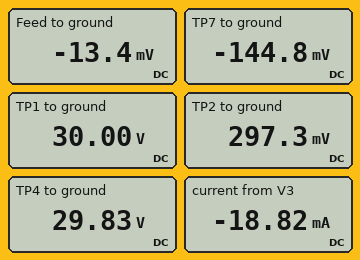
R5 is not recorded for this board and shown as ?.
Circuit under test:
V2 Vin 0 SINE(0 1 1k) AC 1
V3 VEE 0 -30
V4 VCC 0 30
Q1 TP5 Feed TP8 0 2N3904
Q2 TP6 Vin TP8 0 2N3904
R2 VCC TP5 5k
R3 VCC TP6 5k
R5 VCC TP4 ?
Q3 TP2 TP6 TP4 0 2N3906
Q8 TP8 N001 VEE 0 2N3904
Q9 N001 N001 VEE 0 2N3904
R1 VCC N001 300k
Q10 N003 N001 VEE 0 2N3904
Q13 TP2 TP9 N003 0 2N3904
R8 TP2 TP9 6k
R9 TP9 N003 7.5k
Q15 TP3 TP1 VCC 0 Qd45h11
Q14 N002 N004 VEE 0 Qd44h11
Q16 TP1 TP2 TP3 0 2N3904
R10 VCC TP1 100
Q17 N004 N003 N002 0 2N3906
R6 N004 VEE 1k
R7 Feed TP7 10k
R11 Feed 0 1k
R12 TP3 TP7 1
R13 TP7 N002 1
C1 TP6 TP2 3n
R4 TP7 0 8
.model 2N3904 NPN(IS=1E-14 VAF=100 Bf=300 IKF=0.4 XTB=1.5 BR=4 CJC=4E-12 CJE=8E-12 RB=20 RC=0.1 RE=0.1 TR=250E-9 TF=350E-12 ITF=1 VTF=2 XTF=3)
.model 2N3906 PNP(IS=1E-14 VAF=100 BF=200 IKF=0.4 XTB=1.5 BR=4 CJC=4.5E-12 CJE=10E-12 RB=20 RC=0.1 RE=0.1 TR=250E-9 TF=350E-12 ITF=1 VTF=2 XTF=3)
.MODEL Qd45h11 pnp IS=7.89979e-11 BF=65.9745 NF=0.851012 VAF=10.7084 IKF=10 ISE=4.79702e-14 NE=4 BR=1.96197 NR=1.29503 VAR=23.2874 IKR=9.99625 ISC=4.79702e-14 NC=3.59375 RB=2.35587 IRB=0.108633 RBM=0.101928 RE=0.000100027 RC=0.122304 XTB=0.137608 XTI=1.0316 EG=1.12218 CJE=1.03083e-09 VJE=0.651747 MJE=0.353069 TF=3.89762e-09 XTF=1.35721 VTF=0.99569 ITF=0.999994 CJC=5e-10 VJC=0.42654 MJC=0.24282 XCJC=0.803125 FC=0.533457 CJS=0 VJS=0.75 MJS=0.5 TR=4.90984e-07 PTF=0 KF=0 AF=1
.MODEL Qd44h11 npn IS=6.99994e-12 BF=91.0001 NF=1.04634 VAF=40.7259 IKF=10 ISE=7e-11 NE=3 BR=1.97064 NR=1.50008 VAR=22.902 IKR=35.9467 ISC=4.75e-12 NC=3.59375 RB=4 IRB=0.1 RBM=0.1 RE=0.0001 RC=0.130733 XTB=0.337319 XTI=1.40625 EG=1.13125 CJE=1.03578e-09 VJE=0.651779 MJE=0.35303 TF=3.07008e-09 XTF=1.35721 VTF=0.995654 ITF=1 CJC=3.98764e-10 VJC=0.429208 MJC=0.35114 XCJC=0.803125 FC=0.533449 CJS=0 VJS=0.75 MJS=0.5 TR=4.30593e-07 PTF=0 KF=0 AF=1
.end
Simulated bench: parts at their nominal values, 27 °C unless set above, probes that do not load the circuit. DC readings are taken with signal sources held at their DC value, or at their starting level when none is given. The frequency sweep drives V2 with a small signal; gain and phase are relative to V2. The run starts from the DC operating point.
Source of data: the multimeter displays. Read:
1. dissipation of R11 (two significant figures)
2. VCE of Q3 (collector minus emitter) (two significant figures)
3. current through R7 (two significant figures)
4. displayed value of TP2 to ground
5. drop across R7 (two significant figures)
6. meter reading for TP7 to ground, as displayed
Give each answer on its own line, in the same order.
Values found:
180 nW
-30 V
13 µA
297.3 mV
130 mV
-144.8 mV
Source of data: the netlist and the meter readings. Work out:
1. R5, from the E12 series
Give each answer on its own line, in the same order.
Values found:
680 Ω
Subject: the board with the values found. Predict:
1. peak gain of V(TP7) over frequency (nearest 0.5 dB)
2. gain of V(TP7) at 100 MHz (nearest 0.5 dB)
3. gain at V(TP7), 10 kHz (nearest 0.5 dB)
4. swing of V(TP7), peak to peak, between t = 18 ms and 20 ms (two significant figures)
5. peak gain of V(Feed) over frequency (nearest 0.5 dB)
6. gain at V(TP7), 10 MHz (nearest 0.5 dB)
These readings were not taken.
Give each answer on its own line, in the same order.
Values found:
21.0 dB
-46.0 dB
17.5 dB
14 V
0 dB
-16.0 dB
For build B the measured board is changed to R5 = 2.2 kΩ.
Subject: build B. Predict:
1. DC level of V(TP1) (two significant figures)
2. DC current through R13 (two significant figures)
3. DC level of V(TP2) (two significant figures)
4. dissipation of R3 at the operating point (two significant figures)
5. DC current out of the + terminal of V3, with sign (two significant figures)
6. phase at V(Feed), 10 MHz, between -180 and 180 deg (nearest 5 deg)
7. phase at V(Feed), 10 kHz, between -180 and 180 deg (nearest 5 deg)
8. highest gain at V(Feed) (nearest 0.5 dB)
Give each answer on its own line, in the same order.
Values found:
30 V
88 mA
-350 mV
270 µW
-89 mA
40 deg
-100 deg
-0.5 dB
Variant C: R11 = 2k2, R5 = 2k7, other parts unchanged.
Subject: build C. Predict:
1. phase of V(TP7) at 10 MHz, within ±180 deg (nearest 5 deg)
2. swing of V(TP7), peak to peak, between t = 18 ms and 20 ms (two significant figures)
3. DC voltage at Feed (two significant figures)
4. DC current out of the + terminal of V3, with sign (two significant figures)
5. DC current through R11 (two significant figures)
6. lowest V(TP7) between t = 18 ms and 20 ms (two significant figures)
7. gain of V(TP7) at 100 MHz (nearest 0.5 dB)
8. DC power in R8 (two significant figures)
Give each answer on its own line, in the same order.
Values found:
80 deg
1.7 V
-400 mV
-280 mA
180 µA
-5.9 V
-45.5 dB
40 µW
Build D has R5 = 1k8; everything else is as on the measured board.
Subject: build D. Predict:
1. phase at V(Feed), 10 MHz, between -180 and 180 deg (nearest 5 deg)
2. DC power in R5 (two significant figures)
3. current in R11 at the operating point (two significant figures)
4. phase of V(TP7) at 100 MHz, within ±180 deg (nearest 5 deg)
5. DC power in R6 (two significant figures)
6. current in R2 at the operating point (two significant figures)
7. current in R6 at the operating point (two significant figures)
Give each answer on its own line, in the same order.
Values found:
35 deg
110 µW
44 µA
55 deg
370 µW
39 µA
610 µA
